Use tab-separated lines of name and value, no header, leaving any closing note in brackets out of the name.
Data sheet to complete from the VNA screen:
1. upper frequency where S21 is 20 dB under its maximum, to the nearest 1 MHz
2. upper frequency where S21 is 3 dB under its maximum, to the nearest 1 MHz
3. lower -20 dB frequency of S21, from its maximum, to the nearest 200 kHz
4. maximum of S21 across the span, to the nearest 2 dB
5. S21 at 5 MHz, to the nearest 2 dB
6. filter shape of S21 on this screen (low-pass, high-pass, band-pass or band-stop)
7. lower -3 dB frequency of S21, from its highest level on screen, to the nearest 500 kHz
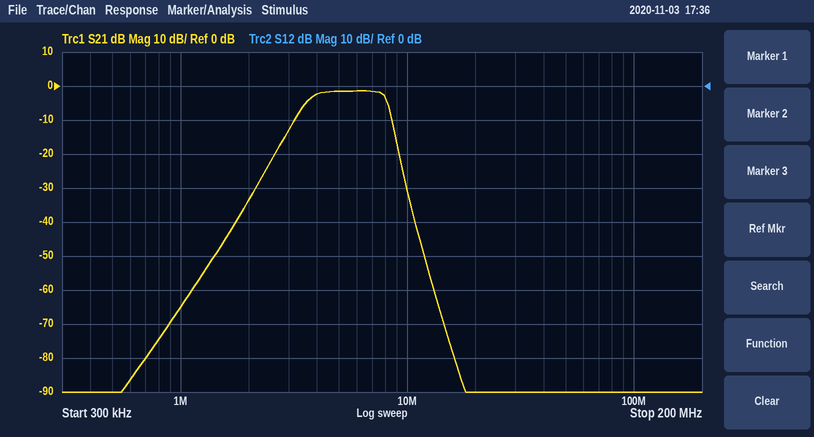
upper frequency where S21 is 20 dB under its maximum, to the nearest 1 MHz	9 MHz
upper frequency where S21 is 3 dB under its maximum, to the nearest 1 MHz	8 MHz
lower -20 dB frequency of S21, from its maximum, to the nearest 200 kHz	2.6 MHz
maximum of S21 across the span, to the nearest 2 dB	-2 dB
S21 at 5 MHz, to the nearest 2 dB	-2 dB
filter shape of S21 on this screen	band-pass
lower -3 dB frequency of S21, from its highest level on screen, to the nearest 500 kHz	3.5 MHz
